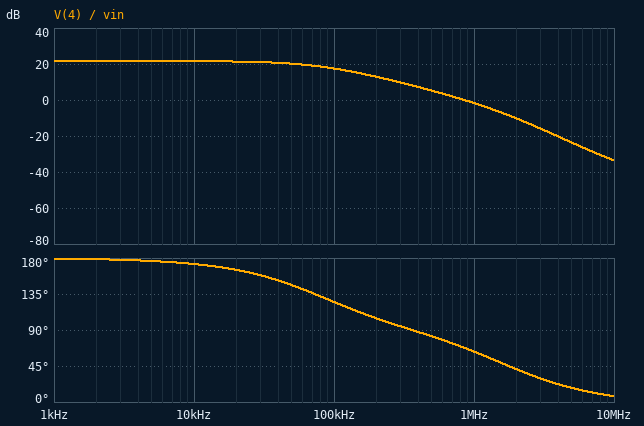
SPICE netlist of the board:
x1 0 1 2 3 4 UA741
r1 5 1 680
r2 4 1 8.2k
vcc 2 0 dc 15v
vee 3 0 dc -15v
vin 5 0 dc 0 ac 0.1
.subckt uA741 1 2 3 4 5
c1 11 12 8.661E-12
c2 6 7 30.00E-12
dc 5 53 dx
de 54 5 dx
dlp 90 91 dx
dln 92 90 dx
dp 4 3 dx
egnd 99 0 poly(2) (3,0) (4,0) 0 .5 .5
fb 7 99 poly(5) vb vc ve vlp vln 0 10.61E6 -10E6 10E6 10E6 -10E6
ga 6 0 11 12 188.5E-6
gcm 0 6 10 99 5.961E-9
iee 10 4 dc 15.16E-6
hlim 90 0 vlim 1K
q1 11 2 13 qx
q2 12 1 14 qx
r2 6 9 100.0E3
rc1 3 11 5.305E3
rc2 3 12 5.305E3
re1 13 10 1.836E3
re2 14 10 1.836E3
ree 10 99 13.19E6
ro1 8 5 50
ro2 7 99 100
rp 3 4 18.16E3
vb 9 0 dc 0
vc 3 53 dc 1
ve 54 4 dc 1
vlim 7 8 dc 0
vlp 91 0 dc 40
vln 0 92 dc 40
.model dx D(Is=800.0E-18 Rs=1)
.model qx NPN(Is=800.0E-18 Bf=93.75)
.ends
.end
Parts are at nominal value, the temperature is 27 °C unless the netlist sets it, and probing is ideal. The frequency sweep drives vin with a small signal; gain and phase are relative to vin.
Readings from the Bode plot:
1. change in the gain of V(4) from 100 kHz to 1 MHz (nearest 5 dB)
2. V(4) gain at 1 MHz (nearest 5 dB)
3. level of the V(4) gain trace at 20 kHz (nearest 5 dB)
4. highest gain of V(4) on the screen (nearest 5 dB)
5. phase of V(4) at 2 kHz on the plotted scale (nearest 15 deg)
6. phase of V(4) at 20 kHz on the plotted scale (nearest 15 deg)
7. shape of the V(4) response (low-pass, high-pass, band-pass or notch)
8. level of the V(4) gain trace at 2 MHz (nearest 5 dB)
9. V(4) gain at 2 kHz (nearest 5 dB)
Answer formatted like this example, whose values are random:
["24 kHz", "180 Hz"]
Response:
["-20 dB", "0 dB", "20 dB", "20 dB", "180 deg", "165 deg", "low-pass", "-10 dB", "20 dB"]
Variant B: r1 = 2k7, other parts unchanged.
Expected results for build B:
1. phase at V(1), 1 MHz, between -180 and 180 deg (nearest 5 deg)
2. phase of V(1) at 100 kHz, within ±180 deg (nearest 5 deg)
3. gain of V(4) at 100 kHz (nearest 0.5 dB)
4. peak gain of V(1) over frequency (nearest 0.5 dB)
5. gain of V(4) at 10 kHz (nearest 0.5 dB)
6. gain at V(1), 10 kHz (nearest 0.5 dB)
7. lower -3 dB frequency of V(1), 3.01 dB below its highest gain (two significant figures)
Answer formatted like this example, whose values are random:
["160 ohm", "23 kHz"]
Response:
["10 deg", "70 deg", "9.0 dB", "-1.5 dB", "9.5 dB", "-30.5 dB", "250 kHz"]
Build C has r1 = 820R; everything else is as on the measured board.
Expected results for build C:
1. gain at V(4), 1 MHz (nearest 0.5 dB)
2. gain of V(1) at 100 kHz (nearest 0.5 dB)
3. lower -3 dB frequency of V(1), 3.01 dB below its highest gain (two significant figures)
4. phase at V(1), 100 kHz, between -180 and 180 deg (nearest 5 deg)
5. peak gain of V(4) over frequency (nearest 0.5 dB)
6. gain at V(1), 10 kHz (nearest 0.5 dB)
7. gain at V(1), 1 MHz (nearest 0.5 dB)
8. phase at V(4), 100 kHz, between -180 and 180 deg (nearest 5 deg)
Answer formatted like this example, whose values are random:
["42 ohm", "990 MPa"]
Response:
["-2.0 dB", "-3.0 dB", "92 kHz", "45 deg", "20.0 dB", "-20.0 dB", "-0.5 dB", "130 deg"]
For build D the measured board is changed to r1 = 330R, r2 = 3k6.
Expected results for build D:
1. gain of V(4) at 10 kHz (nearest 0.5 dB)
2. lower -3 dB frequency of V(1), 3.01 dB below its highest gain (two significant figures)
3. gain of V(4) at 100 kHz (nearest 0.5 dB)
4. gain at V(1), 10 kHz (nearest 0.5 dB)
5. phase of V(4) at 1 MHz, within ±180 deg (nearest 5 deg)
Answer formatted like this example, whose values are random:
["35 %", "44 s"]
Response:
["20.5 dB", "85 kHz", "17.0 dB", "-19.0 dB", "65 deg"]
